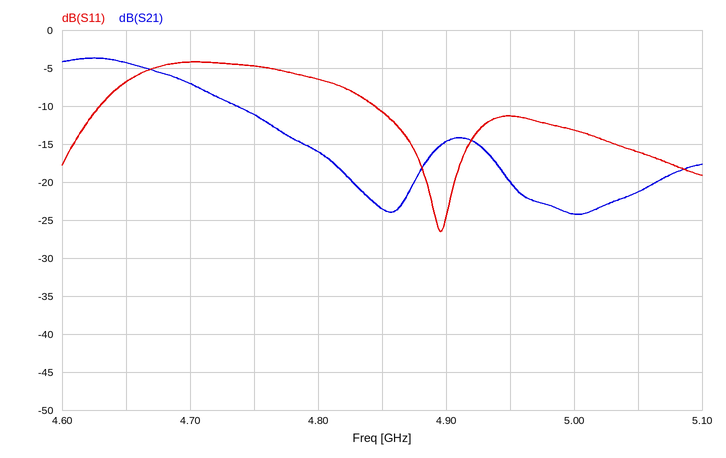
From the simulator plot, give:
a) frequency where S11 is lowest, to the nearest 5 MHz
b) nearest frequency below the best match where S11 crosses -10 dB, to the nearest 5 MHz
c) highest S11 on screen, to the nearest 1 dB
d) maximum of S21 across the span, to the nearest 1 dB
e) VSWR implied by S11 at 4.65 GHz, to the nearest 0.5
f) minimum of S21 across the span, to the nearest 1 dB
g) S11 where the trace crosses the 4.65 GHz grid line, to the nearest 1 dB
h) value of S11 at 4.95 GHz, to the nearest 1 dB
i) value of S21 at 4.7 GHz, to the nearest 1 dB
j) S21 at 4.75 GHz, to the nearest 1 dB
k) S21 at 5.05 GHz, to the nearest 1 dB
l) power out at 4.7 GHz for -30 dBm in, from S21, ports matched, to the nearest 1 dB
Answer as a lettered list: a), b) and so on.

a) 4.895 GHz
b) 4.845 GHz
c) -4 dB
d) -4 dB
e) 2.5
f) -24 dB
g) -7 dB
h) -11 dB
i) -7 dB
j) -11 dB
k) -21 dB
l) -37 dBm
